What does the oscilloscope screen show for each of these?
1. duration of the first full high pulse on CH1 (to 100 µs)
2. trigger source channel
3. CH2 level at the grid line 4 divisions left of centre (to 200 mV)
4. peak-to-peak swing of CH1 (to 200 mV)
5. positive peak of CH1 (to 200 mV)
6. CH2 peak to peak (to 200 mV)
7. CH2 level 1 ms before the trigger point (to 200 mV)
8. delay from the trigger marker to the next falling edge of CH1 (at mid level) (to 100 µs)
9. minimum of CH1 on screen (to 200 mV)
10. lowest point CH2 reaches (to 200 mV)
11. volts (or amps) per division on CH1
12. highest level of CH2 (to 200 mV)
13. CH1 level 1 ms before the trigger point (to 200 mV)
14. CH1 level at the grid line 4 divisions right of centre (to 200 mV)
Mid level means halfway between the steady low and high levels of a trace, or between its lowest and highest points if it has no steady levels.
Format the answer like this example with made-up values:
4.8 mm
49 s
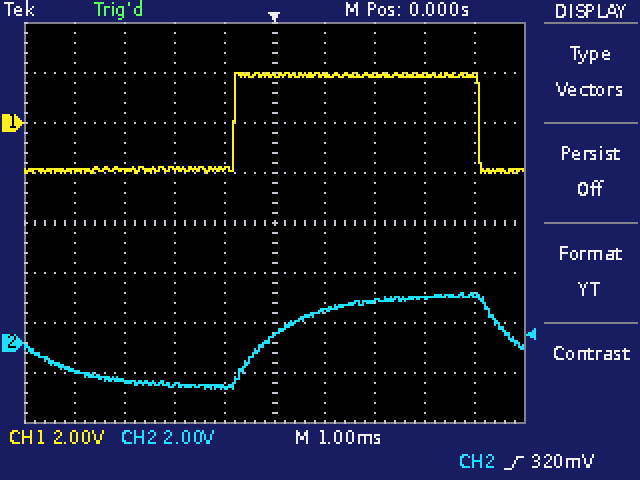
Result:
4.9 ms
CH2
-1.2 V
4.0 V
2.0 V
3.8 V
-1.8 V
4.1 ms
-2.0 V
-1.8 V
2 V
2.0 V
-1.8 V
1.8 V
